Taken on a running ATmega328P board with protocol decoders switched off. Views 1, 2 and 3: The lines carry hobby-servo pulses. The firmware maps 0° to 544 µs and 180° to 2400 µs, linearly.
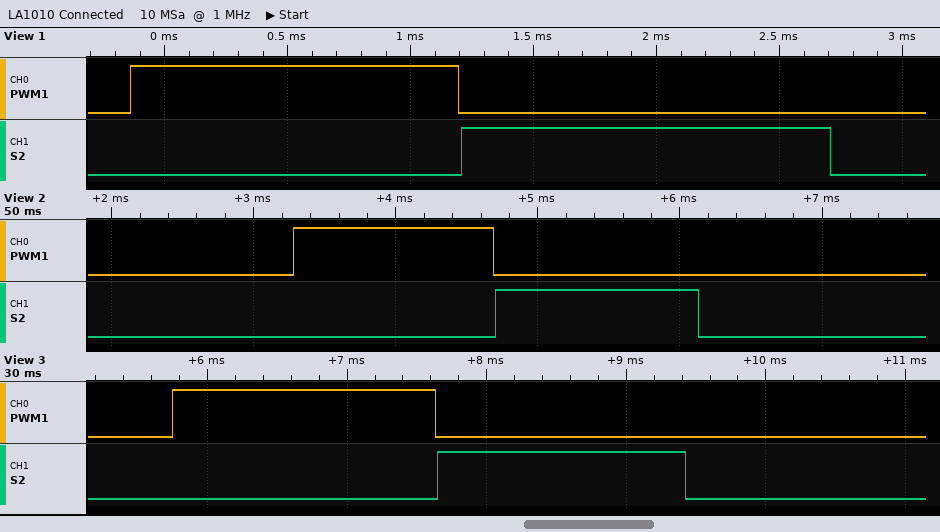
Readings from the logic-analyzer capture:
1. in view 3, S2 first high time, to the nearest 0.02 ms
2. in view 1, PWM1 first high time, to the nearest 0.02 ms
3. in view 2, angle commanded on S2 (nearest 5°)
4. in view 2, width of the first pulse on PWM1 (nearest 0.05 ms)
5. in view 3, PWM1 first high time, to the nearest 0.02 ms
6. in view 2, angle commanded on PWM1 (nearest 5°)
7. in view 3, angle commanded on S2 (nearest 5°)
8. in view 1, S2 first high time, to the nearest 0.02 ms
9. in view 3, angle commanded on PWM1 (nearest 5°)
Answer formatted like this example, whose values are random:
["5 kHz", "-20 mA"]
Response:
["1.78 ms", "1.34 ms", "85°", "1.40 ms", "1.88 ms", "85°", "120°", "1.50 ms", "130°"]
